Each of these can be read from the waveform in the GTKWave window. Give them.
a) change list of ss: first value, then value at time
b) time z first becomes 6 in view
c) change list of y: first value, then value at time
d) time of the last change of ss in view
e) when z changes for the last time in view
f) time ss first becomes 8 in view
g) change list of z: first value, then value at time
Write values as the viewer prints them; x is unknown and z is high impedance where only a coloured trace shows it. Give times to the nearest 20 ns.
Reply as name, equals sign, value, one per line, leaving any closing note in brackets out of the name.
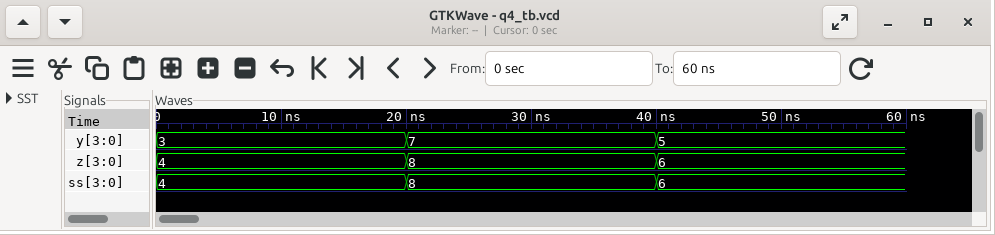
change list of ss: first value, then value at time = 4, 8 at 20 ns, 6 at 40 ns
time z first becomes 6 in view = 40 ns
change list of y: first value, then value at time = 3, 7 at 20 ns, 5 at 40 ns
time of the last change of ss in view = 40 ns
when z changes for the last time in view = 40 ns
time ss first becomes 8 in view = 20 ns
change list of z: first value, then value at time = 4, 8 at 20 ns, 6 at 40 ns
